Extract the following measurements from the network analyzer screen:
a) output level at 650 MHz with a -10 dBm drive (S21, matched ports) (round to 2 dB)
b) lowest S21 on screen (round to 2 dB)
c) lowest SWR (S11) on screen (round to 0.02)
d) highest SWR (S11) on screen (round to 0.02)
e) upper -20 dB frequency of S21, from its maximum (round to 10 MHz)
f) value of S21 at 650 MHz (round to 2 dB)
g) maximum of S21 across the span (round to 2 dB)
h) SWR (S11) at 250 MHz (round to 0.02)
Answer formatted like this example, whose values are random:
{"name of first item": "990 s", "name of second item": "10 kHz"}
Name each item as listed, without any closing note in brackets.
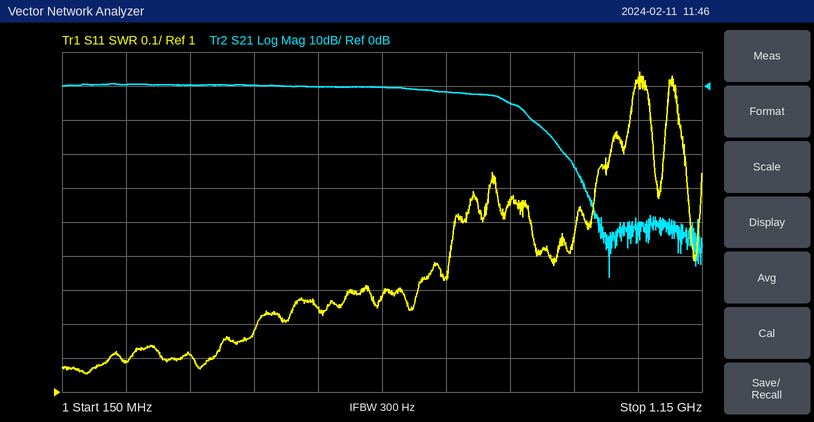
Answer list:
{"output level at 650 MHz with a -10 dBm drive (S21, matched ports)": "-10 dBm", "lowest S21 on screen": "-56 dB", "lowest SWR (S11) on screen": "1.06", "highest SWR (S11) on screen": "1.94", "upper -20 dB frequency of S21, from its maximum": "930 MHz", "value of S21 at 650 MHz": "0 dB", "maximum of S21 across the span": "0 dB", "SWR (S11) at 250 MHz": "1.08"}
